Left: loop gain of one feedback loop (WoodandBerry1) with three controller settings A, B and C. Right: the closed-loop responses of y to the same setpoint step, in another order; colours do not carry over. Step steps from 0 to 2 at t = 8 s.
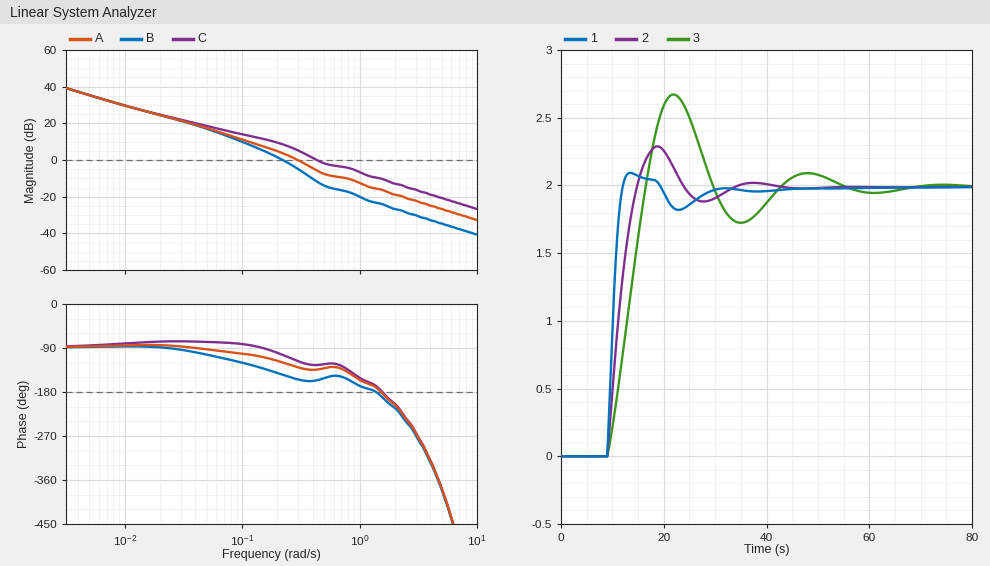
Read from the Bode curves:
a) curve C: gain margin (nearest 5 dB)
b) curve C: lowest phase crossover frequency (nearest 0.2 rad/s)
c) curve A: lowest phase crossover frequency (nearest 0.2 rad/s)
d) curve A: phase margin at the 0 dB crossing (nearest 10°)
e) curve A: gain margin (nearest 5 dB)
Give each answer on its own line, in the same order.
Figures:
10 dB
1.6 rad/s
1.6 rad/s
50°
15 dB
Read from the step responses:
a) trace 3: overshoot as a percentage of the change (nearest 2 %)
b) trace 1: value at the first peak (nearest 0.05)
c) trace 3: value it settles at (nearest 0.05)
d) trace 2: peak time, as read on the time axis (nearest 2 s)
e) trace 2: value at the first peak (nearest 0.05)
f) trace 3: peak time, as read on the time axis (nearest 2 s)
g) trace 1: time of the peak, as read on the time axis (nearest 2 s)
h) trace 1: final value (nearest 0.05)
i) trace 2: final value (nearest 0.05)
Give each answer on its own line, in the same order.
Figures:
34 %
2.10
2.00
18 s
2.30
22 s
14 s
2.00
2.00
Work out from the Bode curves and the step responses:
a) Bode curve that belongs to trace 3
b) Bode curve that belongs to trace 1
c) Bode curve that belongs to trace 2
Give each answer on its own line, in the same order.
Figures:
B
C
A
